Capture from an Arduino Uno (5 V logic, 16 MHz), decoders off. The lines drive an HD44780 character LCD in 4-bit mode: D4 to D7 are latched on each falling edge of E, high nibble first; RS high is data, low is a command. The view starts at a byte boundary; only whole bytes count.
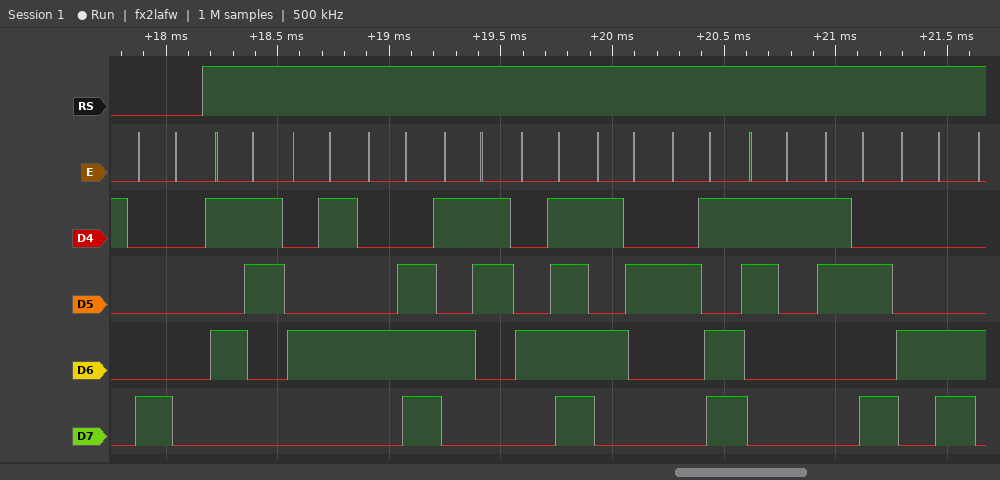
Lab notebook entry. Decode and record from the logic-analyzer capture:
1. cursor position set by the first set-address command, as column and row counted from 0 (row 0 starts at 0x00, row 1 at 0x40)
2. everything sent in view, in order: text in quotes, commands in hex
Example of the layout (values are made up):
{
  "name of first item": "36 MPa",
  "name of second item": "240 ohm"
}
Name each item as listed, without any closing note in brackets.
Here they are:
{
  "cursor position set by the first set-address command, as column and row counted from 0": "column 0, row 0",
  "everything sent in view, in order: text in quotes, commands in hex": "0x80 \"SENSOR-1:L\""
}
